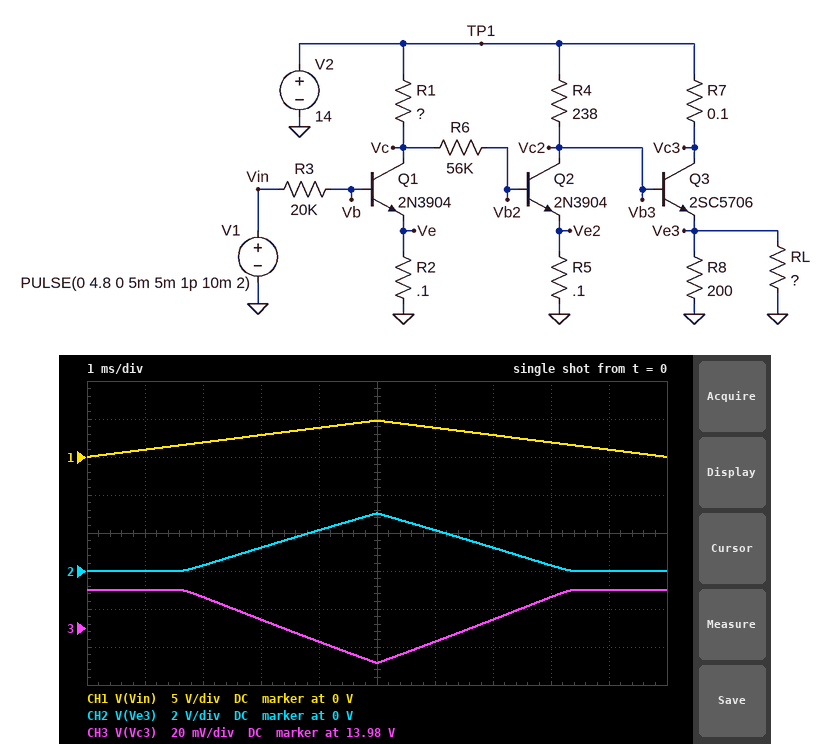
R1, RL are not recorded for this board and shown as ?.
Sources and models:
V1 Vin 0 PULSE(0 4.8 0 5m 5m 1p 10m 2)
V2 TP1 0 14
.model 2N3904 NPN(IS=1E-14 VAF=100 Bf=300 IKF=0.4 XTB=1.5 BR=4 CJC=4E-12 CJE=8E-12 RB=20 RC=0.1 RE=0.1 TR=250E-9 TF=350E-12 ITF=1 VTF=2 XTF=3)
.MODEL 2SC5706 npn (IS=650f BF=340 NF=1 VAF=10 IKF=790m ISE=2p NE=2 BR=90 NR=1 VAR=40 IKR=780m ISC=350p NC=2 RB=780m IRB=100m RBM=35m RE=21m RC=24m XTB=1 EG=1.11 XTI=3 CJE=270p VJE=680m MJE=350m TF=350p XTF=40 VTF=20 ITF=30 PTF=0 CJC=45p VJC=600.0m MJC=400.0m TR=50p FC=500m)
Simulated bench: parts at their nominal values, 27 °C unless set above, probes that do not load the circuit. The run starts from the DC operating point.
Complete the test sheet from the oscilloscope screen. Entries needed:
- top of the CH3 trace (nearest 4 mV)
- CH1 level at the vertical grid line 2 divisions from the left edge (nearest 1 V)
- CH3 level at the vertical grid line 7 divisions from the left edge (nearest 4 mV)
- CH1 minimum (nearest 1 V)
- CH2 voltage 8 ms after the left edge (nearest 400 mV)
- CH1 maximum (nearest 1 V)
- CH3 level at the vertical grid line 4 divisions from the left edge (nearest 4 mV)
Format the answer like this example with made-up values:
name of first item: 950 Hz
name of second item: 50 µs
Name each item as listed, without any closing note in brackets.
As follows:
top of the CH3 trace: 14.000 V
CH1 level at the vertical grid line 2 divisions from the left edge: 2 V
CH3 level at the vertical grid line 7 divisions from the left edge: 13.984 V
CH1 minimum: 0 V
CH2 voltage 8 ms after the left edge: 400 mV
CH1 maximum: 5 V
CH3 level at the vertical grid line 4 divisions from the left edge: 13.972 V
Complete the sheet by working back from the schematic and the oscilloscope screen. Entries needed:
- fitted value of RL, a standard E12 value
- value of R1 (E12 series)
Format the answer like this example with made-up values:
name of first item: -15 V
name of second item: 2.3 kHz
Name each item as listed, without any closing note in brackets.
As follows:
fitted value of RL, a standard E12 value: 8.2 Ω
value of R1: 82 Ω
